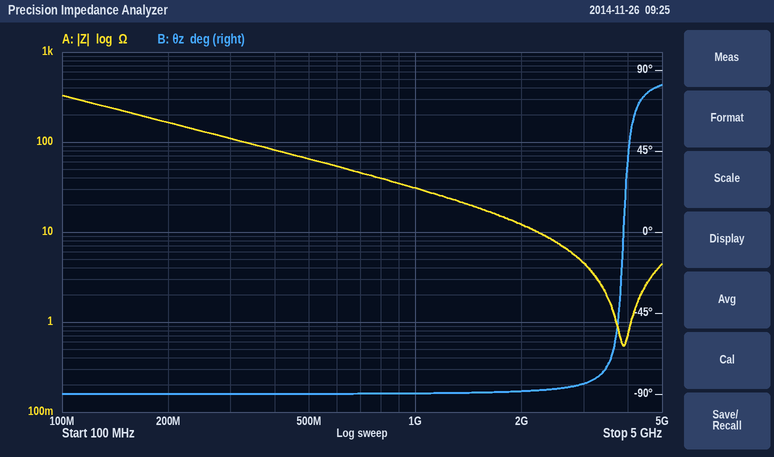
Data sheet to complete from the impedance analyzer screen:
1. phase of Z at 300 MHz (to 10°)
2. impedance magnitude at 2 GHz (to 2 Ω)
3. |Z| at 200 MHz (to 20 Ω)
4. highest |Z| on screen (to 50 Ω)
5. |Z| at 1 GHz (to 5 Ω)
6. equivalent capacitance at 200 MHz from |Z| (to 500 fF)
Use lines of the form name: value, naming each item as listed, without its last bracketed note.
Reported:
phase of Z at 300 MHz: -90°
impedance magnitude at 2 GHz: 12 Ω
|Z| at 200 MHz: 160 Ω
highest |Z| on screen: 350 Ω
|Z| at 1 GHz: 30 Ω
equivalent capacitance at 200 MHz from |Z|: 5.0 pF
